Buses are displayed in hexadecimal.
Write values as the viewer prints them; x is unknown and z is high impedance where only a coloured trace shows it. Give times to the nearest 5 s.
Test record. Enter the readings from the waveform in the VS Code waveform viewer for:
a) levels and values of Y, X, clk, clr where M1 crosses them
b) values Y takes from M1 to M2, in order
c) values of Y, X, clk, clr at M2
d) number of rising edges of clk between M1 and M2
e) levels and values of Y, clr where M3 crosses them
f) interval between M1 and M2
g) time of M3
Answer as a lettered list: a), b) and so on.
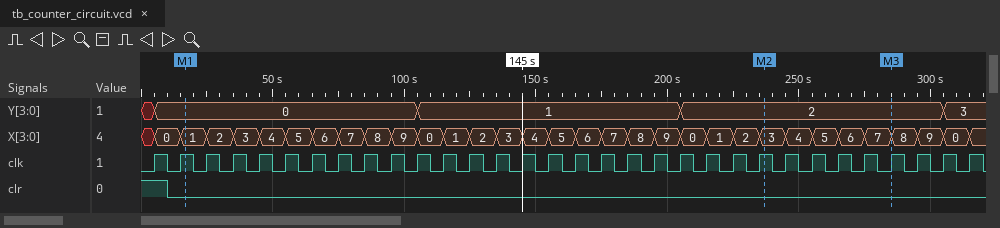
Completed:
a) Y=0, X=1, clk=1, clr=0
b) 0, 1, 2
c) Y=2, X=3, clk=1, clr=0
d) 22
e) Y=2, clr=0
f) 220 s
g) 285 s
